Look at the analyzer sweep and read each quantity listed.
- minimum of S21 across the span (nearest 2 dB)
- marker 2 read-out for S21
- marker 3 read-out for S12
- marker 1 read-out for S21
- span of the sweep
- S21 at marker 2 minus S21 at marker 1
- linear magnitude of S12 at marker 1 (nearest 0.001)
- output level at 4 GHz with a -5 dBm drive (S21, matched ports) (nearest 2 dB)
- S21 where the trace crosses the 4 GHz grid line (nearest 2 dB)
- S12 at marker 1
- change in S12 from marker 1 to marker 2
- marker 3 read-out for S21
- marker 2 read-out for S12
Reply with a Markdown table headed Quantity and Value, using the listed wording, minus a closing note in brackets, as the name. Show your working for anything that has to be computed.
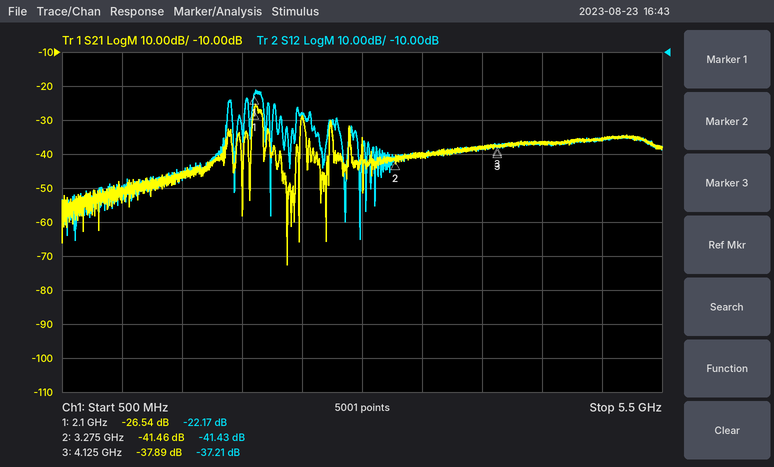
| Quantity | Value |
|---|---|
| minimum of S21 across the span | -72 dB |
| marker 2 read-out for S21 | -41.46 dB |
| marker 3 read-out for S12 | -37.21 dB |
| marker 1 read-out for S21 | -26.54 dB |
| span of the sweep | 5 GHz |
| S21 at marker 2 minus S21 at marker 1 | -41.46 − (-26.54) = -14.92 dB |
| linear magnitude of S12 at marker 1 | 10^(-22.17/20) ≈ 0.078 |
| output level at 4 GHz with a -5 dBm drive (S21, matched ports) | -5 dBm + (-38 dB) = -44 dBm |
| S21 where the trace crosses the 4 GHz grid line | -38 dB |
| S12 at marker 1 | -22.17 dB |
| change in S12 from marker 1 to marker 2 | -41.43 − (-22.17) = -19.26 dB |
| marker 3 read-out for S21 | -37.89 dB |
| marker 2 read-out for S12 | -41.43 dB |
